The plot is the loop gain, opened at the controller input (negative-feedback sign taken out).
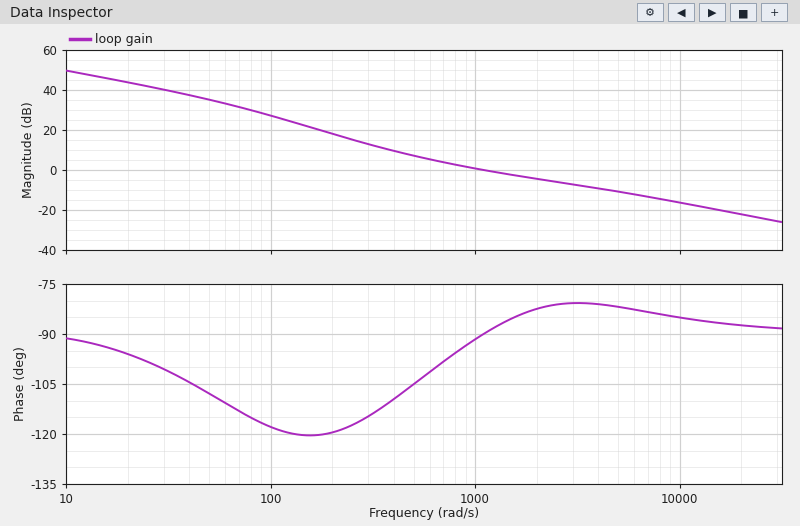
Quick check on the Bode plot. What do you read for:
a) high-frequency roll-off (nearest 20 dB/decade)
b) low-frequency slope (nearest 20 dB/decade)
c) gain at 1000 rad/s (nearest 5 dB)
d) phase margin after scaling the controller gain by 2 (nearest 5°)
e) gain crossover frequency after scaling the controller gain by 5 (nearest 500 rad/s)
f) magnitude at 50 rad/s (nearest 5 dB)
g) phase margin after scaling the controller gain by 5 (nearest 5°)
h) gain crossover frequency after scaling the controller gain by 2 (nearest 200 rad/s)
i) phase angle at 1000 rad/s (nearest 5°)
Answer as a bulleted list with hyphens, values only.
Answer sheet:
- -20 dB/decade
- -20 dB/decade
- 0 dB
- 100°
- 7500 rad/s
- 35 dB
- 95°
- 2600 rad/s
- -90°
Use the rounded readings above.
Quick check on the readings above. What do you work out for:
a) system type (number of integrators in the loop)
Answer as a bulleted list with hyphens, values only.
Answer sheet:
- 1
